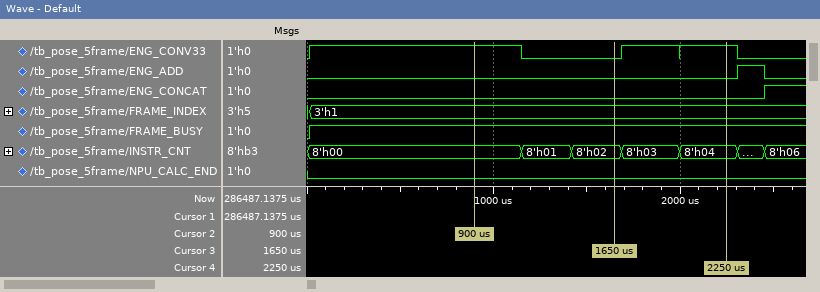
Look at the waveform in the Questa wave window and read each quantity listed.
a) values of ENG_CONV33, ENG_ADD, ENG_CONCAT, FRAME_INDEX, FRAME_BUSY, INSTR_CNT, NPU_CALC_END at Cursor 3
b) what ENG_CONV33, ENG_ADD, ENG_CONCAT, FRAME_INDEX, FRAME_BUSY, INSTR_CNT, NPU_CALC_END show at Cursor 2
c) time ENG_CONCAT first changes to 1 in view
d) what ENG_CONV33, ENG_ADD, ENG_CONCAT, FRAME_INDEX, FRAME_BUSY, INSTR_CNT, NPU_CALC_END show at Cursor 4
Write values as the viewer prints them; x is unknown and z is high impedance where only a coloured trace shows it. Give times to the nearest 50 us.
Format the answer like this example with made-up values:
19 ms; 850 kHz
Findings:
ENG_CONV33=0, ENG_ADD=0, ENG_CONCAT=0, FRAME_INDEX=3'h1, FRAME_BUSY=1, INSTR_CNT=8'h02, NPU_CALC_END=0; ENG_CONV33=1, ENG_ADD=0, ENG_CONCAT=0, FRAME_INDEX=3'h1, FRAME_BUSY=1, INSTR_CNT=8'h00, NPU_CALC_END=0; 2450 us; ENG_CONV33=1, ENG_ADD=0, ENG_CONCAT=0, FRAME_INDEX=3'h1, FRAME_BUSY=1, INSTR_CNT=8'h04, NPU_CALC_END=0
